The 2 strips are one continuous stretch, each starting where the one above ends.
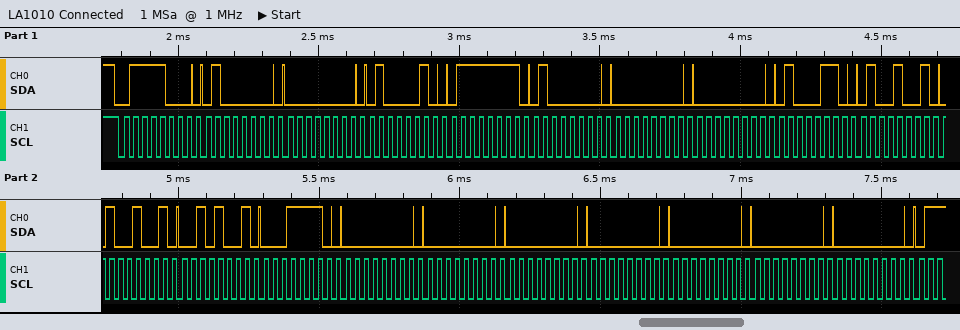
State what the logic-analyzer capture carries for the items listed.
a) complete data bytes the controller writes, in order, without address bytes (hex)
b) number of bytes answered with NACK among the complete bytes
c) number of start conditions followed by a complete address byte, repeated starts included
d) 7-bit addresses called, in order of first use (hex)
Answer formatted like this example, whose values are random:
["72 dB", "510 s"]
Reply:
["40 00 42 7F 40 00 00 46 49 49 29 1E 00 00 00 00 00 00 00", "0", "1", "0x3C"]
